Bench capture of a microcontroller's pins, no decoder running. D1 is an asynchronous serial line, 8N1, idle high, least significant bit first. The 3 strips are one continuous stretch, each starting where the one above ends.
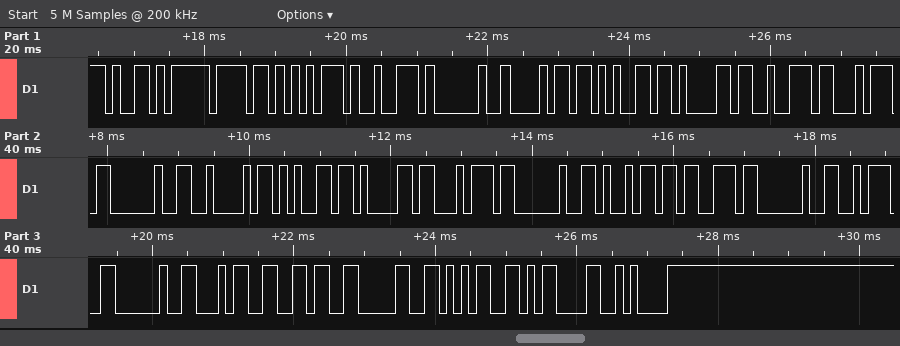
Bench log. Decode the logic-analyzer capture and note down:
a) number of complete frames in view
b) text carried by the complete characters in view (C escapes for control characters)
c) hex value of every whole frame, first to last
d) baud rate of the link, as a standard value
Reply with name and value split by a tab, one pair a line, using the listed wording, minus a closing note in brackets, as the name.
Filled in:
number of complete frames in view	27
text carried by the complete characters in view	"Your heart Beat is : 4605\r\n"
hex value of every whole frame, first to last	59 6F 75 72 20 68 65 61 72 74 20 42 65 61 74 20 69 73 20 3A 20 34 36 30 35 0D 0A
baud rate of the link, as a standard value	9600 baud
